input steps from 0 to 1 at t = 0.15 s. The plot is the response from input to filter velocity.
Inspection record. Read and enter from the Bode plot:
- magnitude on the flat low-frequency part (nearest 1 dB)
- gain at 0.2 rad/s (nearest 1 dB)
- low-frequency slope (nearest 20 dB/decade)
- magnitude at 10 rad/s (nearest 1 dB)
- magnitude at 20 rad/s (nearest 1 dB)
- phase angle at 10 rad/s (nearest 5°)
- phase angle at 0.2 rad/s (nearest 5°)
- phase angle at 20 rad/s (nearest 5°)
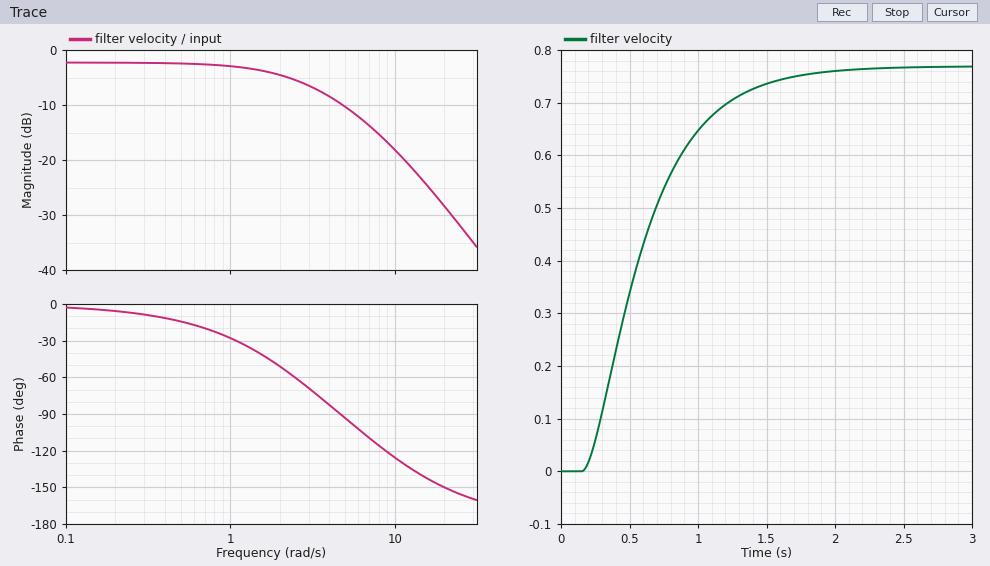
-2 dB
-2 dB
0 dB/decade
-18 dB
-28 dB
-125°
-5°
-150°
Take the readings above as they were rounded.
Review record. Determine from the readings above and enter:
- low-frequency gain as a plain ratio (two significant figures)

0.79
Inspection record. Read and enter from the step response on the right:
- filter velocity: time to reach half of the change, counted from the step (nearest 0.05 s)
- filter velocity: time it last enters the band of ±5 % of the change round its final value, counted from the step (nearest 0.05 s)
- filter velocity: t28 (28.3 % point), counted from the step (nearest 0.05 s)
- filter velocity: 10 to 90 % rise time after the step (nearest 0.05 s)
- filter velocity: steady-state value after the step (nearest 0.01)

0.40 s
1.30 s
0.25 s
0.90 s
0.77
